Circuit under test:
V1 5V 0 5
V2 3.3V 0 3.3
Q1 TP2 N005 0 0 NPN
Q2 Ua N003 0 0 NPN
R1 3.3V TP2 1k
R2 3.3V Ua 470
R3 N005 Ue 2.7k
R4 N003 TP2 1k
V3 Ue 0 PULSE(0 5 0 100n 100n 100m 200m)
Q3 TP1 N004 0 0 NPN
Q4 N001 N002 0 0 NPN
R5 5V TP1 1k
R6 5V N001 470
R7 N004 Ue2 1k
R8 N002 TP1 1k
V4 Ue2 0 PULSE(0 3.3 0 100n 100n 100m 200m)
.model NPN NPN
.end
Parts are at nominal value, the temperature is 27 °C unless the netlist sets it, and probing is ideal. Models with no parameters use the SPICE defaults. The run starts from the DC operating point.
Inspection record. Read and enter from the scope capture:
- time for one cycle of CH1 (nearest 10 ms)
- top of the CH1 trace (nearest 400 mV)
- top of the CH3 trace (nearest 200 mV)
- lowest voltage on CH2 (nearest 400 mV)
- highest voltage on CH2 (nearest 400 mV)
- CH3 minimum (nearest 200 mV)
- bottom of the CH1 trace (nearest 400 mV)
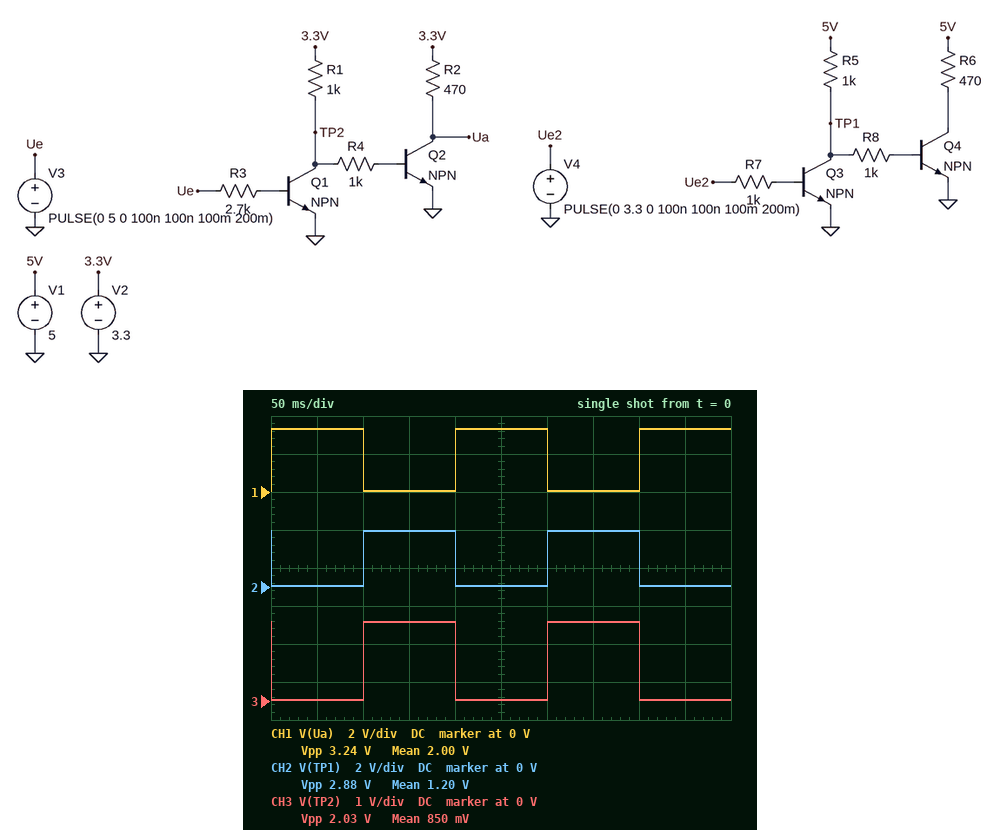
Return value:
200 ms
3.2 V
2.0 V
0 V
2.8 V
0 V
0 V
